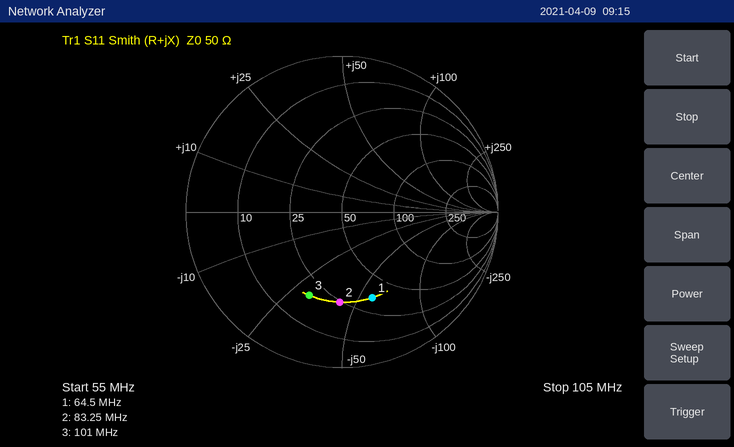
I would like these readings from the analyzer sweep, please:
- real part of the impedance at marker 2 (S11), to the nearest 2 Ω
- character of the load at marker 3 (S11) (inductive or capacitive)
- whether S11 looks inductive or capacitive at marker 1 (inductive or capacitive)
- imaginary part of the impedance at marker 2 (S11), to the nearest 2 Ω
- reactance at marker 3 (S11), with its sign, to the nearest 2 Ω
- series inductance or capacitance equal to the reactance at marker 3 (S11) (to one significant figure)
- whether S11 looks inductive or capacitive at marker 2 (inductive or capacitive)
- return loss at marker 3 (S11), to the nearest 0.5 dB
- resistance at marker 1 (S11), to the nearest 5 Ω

24 Ω
capacitive
capacitive
-42 Ω
-30 Ω
50 pF
capacitive
5.0 dB
35 Ω
